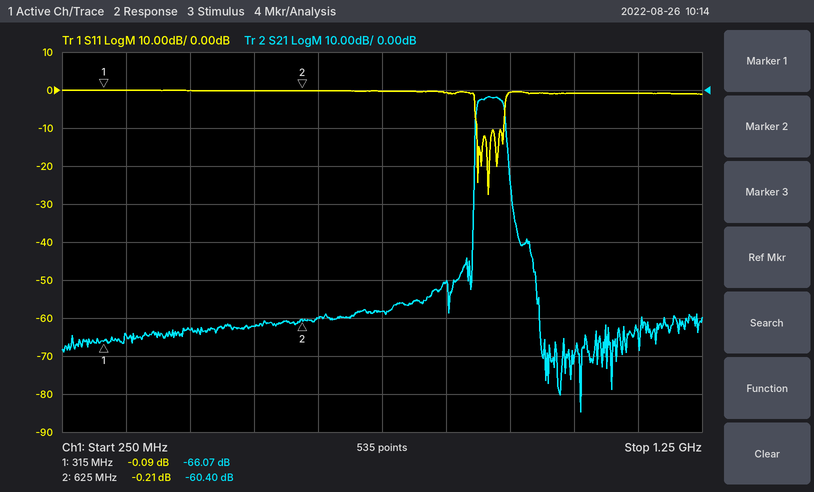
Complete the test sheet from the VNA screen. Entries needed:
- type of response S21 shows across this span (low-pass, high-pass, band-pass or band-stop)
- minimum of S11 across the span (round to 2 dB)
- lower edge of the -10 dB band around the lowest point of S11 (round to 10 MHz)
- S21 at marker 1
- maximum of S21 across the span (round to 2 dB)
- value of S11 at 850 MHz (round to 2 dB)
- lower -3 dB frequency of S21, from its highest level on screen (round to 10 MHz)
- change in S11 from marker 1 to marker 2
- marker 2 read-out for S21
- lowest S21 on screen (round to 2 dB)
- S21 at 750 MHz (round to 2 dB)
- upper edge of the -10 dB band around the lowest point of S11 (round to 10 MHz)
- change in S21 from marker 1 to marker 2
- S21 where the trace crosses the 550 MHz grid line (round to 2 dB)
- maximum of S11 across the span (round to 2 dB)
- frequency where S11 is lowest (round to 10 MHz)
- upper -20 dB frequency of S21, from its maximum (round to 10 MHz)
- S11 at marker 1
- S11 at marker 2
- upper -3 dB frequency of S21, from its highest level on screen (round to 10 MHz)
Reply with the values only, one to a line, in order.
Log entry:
band-pass
-28 dB
900 MHz
-66.07 dB
-2 dB
0 dB
900 MHz
-0.12 dB
-60.40 dB
-84 dB
-58 dB
940 MHz
5.67 dB
-62 dB
0 dB
920 MHz
950 MHz
-0.09 dB
-0.21 dB
940 MHz
